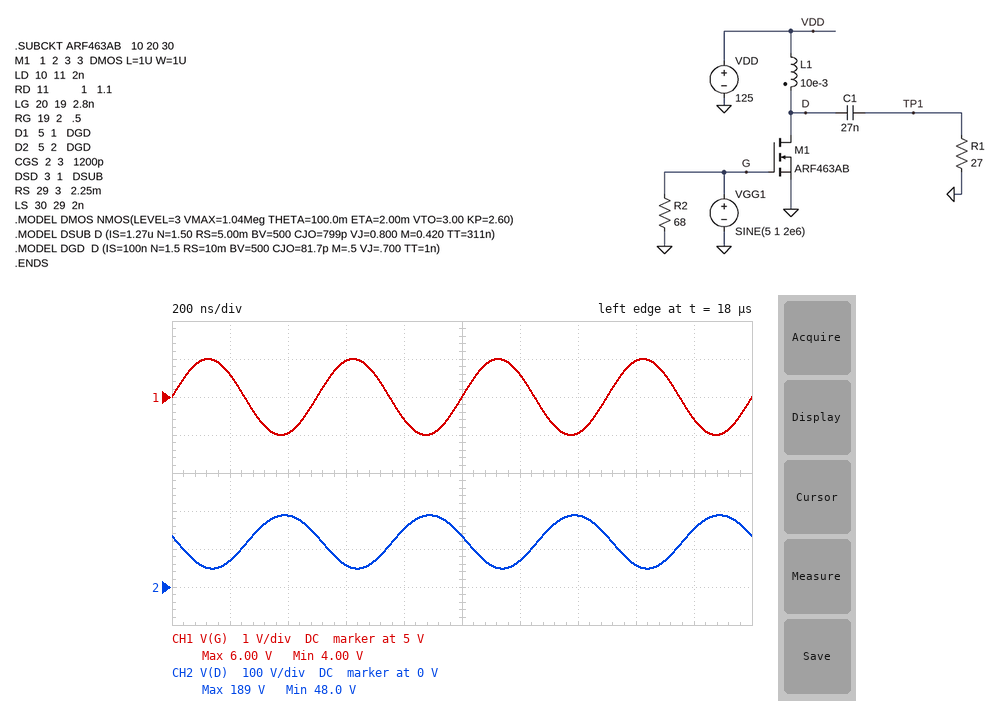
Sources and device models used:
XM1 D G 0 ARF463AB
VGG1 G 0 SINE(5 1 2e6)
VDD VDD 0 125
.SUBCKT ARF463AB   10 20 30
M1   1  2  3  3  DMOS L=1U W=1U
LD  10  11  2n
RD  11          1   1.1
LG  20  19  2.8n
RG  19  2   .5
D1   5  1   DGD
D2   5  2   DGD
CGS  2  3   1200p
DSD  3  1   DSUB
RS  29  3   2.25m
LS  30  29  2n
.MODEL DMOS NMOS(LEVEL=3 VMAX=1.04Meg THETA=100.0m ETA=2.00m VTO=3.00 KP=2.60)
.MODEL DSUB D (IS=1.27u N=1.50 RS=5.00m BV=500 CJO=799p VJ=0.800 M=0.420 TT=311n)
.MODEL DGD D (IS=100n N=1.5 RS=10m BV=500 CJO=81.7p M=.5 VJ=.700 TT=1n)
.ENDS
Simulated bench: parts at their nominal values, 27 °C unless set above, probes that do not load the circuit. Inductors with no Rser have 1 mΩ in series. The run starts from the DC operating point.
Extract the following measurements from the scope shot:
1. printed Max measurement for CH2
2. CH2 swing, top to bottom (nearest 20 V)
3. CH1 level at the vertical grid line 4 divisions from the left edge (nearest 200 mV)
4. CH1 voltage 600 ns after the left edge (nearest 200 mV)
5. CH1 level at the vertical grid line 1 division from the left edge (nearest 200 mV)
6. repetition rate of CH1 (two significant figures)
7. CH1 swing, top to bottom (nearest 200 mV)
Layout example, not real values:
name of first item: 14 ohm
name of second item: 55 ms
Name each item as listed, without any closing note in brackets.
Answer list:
printed Max measurement for CH2: 189 V
CH2 swing, top to bottom: 140 V
CH1 level at the vertical grid line 4 divisions from the left edge: 4.4 V
CH1 voltage 600 ns after the left edge: 6.0 V
CH1 level at the vertical grid line 1 division from the left edge: 5.6 V
repetition rate of CH1: 2.0 MHz
CH1 swing, top to bottom: 2.0 V
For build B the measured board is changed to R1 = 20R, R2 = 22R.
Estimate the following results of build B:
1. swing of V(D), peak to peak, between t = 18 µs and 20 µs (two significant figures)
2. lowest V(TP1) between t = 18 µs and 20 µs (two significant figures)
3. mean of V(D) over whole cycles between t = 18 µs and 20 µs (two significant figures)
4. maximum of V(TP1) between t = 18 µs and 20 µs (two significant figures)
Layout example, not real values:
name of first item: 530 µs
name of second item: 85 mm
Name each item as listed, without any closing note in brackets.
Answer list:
swing of V(D), peak to peak, between t = 18 µs and 20 µs: 110 V
lowest V(TP1) between t = 18 µs and 20 µs: -58 V
mean of V(D) over whole cycles between t = 18 µs and 20 µs: 120 V
maximum of V(TP1) between t = 18 µs and 20 µs: 55 V
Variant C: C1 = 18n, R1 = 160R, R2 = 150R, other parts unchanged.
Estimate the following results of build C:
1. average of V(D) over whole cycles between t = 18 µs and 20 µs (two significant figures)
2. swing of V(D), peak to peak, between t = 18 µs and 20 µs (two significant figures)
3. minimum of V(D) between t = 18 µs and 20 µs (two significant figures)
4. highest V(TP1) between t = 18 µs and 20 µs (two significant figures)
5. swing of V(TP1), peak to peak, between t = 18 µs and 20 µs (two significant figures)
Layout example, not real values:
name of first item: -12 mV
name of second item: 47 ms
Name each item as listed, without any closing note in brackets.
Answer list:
average of V(D) over whole cycles between t = 18 µs and 20 µs: 130 V
swing of V(D), peak to peak, between t = 18 µs and 20 µs: 270 V
minimum of V(D) between t = 18 µs and 20 µs: 9.2 V
highest V(TP1) between t = 18 µs and 20 µs: 150 V
swing of V(TP1), peak to peak, between t = 18 µs and 20 µs: 280 V
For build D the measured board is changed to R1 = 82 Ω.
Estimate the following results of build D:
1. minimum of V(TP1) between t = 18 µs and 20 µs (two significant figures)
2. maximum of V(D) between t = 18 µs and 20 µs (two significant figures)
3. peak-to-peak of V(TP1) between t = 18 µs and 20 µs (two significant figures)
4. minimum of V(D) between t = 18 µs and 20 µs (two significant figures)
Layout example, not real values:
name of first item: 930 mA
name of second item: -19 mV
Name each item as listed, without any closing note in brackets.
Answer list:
minimum of V(TP1) between t = 18 µs and 20 µs: -120 V
maximum of V(D) between t = 18 µs and 20 µs: 250 V
peak-to-peak of V(TP1) between t = 18 µs and 20 µs: 240 V
minimum of V(D) between t = 18 µs and 20 µs: 10 V
